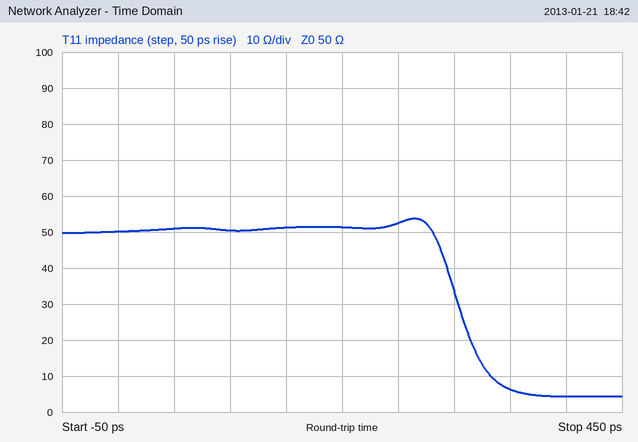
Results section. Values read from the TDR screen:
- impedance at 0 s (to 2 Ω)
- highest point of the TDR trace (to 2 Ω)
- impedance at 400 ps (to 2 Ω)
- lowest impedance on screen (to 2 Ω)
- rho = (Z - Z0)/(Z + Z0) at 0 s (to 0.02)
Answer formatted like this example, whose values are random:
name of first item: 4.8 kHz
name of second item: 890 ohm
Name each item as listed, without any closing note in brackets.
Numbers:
impedance at 0 s: 50 Ω
highest point of the TDR trace: 54 Ω
impedance at 400 ps: 4 Ω
lowest impedance on screen: 4 Ω
rho = (Z - Z0)/(Z + Z0) at 0 s: 0.00
